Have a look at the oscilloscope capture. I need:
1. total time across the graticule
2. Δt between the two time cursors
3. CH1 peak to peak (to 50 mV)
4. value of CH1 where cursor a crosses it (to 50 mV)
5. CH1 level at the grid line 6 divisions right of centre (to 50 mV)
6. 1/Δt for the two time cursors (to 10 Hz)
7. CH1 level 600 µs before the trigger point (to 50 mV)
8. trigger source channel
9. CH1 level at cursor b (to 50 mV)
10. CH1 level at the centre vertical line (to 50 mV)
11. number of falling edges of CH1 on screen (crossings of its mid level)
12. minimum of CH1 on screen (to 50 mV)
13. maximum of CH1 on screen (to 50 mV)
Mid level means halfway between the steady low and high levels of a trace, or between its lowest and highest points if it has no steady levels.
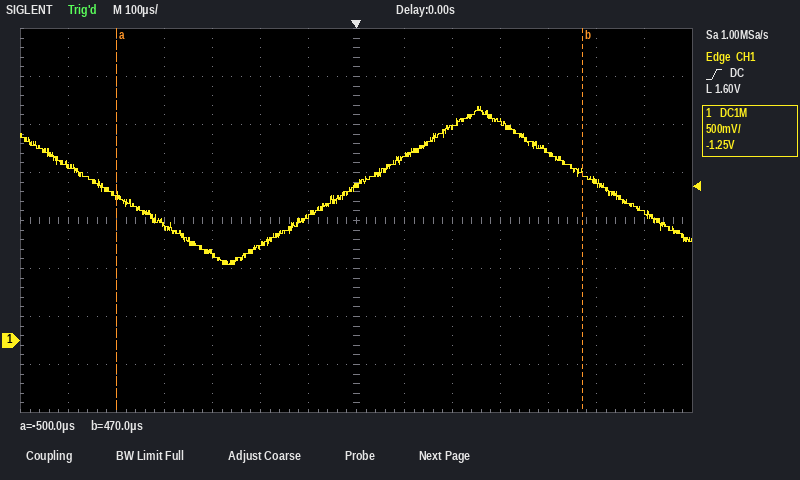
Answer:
1.4 ms
970 µs
1.65 V
1.50 V
1.35 V
1.03 kHz
1.85 V
CH1
1.75 V
1.60 V
2
800 mV
2.45 V
